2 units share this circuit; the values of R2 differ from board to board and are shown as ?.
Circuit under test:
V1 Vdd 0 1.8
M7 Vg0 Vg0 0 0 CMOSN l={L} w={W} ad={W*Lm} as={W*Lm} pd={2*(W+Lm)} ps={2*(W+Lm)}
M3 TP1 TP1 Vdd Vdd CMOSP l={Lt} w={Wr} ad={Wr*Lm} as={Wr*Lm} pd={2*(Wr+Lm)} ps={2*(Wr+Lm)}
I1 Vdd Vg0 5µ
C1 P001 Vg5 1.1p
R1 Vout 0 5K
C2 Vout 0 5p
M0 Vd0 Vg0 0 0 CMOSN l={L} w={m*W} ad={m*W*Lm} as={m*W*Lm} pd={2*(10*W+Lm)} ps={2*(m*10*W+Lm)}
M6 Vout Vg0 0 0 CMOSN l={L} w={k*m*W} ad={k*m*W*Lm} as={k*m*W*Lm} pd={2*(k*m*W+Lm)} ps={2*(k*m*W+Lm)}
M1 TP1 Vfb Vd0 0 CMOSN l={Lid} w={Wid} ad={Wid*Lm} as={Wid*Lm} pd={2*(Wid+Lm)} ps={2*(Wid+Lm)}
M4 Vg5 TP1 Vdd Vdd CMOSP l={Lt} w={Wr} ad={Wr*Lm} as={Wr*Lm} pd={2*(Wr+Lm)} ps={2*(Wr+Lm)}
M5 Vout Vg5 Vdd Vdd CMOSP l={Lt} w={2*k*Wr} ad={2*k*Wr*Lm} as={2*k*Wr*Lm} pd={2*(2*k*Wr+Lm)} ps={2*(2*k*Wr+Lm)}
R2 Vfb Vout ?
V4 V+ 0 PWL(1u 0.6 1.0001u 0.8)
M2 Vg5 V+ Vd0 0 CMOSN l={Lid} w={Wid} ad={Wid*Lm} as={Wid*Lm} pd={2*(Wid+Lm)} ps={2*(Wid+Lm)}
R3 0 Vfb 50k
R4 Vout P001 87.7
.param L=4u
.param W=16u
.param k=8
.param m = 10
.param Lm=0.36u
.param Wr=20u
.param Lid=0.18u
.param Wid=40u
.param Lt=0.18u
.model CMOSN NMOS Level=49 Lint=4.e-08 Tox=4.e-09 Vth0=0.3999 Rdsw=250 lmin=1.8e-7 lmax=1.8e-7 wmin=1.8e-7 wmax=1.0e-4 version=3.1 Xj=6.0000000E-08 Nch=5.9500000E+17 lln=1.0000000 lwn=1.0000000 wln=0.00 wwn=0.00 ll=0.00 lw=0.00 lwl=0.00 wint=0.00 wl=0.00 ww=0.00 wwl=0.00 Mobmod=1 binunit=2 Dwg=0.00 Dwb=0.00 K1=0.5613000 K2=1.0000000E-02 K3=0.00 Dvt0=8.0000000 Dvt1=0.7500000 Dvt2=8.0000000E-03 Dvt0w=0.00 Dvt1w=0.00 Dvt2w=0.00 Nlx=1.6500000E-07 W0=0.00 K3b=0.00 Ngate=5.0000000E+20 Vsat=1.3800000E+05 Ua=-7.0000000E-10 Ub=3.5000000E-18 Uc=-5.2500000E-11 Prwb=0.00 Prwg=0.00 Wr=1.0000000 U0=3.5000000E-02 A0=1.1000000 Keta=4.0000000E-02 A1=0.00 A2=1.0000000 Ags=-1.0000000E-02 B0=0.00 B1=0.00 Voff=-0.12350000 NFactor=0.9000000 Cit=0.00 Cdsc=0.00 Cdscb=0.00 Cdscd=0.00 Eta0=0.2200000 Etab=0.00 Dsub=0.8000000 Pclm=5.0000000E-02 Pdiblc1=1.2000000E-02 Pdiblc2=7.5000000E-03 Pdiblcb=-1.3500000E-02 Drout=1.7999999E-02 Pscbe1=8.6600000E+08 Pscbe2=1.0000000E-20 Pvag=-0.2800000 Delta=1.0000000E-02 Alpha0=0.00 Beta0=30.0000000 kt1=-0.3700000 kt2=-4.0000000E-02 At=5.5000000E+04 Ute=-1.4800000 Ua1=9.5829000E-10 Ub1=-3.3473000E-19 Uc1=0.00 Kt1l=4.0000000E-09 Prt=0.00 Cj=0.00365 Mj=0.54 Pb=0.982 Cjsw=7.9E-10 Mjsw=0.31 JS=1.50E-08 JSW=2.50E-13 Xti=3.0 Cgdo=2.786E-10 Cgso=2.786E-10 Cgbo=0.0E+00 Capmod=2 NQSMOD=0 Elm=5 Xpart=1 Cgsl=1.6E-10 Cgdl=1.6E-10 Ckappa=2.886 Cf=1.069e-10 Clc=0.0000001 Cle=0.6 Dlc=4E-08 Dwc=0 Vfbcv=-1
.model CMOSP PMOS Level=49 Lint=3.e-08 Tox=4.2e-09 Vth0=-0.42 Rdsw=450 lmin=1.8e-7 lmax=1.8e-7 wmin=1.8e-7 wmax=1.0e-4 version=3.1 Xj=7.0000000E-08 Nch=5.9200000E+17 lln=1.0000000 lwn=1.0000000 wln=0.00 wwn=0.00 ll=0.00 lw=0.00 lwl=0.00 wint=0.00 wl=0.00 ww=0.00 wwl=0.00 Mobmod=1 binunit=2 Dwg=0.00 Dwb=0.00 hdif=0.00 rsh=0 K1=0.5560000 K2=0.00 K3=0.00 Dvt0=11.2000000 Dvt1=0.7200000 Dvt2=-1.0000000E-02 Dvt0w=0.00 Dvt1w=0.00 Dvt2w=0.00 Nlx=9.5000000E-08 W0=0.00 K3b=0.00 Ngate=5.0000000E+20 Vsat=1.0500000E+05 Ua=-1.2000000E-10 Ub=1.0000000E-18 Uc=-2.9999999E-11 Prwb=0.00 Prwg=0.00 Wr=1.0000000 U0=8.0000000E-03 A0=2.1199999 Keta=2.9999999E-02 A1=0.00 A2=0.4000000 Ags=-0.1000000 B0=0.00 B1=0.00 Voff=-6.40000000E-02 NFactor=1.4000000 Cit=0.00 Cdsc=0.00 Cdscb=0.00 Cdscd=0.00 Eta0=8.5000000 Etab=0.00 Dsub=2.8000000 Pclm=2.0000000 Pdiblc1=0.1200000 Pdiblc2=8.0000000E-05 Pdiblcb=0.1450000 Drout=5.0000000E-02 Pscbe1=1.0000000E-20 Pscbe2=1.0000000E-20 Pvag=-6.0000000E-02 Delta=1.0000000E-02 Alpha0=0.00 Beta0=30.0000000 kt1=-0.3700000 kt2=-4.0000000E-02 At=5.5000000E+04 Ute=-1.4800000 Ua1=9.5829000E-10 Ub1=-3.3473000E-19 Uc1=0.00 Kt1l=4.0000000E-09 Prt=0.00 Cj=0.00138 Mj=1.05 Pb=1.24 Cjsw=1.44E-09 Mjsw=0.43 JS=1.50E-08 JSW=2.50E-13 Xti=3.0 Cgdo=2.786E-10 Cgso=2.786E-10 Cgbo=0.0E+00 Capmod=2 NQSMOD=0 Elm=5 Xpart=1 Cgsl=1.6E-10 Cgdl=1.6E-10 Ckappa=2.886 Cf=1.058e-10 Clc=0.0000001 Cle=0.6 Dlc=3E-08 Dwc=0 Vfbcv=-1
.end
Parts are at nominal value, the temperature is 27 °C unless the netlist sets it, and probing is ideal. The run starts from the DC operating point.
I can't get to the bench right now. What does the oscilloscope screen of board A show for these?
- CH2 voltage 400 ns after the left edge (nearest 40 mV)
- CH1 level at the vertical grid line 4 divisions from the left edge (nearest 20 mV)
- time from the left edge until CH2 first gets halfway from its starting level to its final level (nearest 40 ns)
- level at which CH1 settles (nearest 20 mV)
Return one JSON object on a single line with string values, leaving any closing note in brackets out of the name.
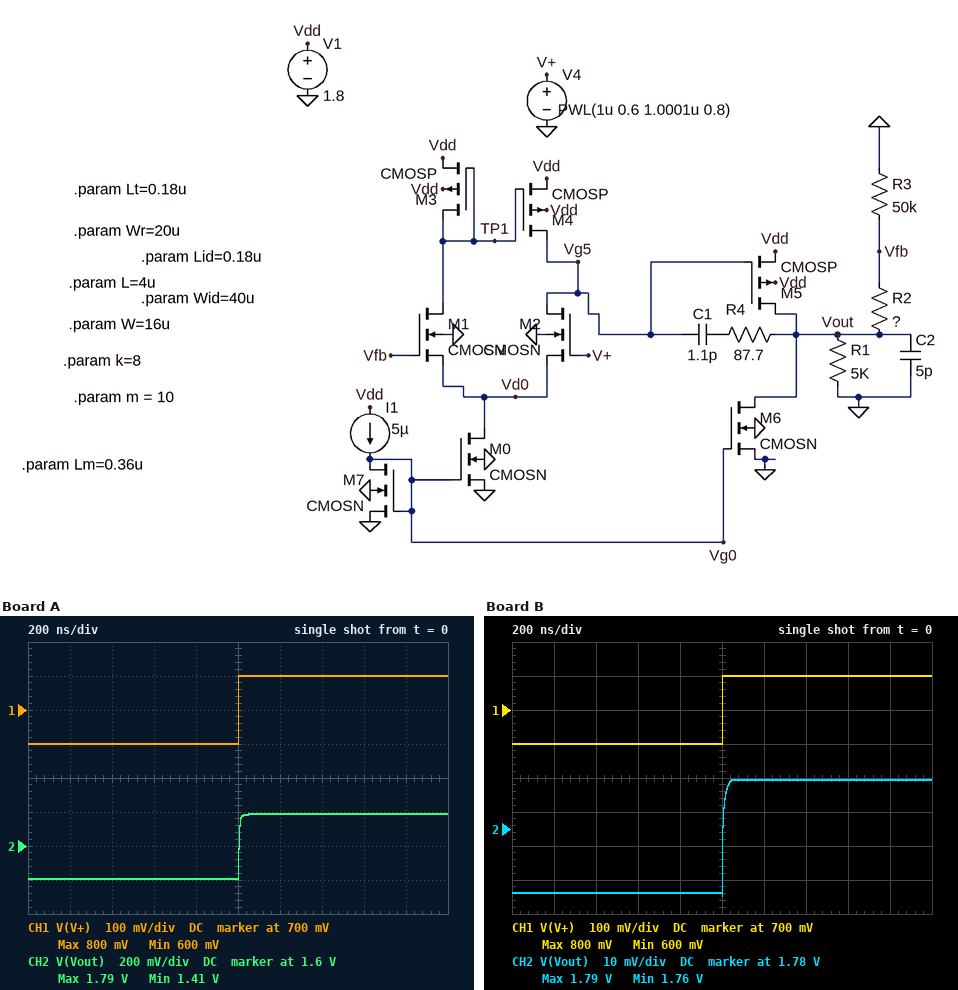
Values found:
{"CH2 voltage 400 ns after the left edge": "1.40 V", "CH1 level at the vertical grid line 4 divisions from the left edge": "600 mV", "time from the left edge until CH2 first gets halfway from its starting level to its final level": "1.00 µs", "level at which CH1 settles": "800 mV"}
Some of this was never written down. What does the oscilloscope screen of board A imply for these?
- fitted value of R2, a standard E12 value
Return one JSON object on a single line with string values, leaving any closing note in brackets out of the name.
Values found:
{"fitted value of R2, a standard E12 value": "68 kΩ"}
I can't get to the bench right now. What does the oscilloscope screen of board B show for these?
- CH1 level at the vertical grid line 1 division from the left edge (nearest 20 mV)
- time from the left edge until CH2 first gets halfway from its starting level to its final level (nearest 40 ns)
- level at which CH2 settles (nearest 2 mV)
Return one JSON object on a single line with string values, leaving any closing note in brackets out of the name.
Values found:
{"CH1 level at the vertical grid line 1 division from the left edge": "600 mV", "time from the left edge until CH2 first gets halfway from its starting level to its final level": "1.00 µs", "level at which CH2 settles": "1.794 V"}
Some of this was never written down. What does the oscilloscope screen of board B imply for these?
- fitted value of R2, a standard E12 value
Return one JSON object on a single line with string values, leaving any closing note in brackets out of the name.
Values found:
{"fitted value of R2, a standard E12 value": "100 kΩ"}
